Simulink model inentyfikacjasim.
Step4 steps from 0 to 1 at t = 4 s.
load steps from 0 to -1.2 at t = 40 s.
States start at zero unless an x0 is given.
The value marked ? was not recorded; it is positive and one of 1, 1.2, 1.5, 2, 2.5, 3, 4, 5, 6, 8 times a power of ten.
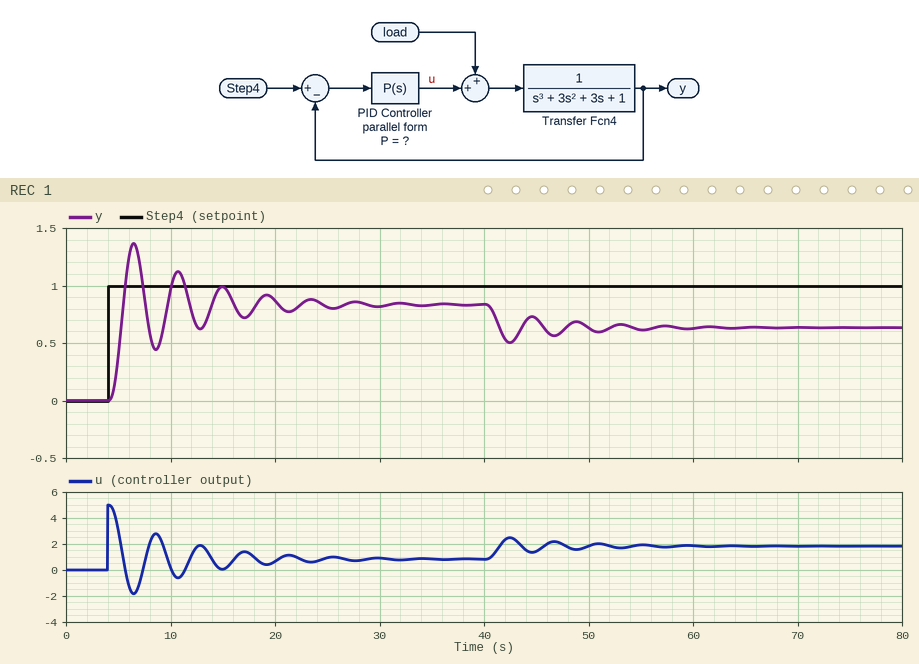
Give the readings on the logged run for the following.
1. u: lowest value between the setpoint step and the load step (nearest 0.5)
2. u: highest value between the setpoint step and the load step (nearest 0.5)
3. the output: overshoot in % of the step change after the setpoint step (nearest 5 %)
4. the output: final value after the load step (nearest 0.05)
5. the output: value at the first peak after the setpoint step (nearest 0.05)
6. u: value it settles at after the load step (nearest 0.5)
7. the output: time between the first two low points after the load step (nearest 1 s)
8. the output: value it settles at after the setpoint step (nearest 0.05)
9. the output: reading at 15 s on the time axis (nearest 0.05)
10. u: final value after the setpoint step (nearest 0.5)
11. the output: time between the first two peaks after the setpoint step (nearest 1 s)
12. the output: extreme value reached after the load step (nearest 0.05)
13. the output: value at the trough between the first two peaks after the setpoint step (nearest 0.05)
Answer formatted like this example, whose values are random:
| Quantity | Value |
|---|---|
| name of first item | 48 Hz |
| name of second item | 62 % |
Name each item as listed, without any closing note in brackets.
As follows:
| Quantity | Value |
|---|---|
| u: lowest value between the setpoint step and the load step | -2.0 |
| u: highest value between the setpoint step and the load step | 5.0 |
| the output: overshoot in % of the step change after the setpoint step | 65 % |
| the output: final value after the load step | 0.65 |
| the output: value at the first peak after the setpoint step | 1.35 |
| u: value it settles at after the load step | 2.0 |
| the output: time between the first two low points after the load step | 4 s |
| the output: value it settles at after the setpoint step | 0.85 |
| the output: reading at 15 s on the time axis | 1.00 |
| u: final value after the setpoint step | 1.0 |
| the output: time between the first two peaks after the setpoint step | 4 s |
| the output: extreme value reached after the load step | 0.50 |
| the output: value at the trough between the first two peaks after the setpoint step | 0.45 |
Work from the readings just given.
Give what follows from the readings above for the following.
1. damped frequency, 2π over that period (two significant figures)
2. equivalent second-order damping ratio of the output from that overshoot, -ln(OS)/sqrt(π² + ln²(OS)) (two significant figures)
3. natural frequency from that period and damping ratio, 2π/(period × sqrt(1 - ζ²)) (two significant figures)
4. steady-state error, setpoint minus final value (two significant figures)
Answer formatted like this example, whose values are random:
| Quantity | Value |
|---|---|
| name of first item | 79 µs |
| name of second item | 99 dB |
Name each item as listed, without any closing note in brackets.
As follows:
| Quantity | Value |
|---|---|
| damped frequency, 2π over that period | 1.6 rad/s |
| equivalent second-order damping ratio of the output from that overshoot, -ln(OS)/sqrt(π² + ln²(OS)) | 0.14 |
| natural frequency from that period and damping ratio, 2π/(period × sqrt(1 - ζ²)) | 1.6 rad/s |
| steady-state error, setpoint minus final value | 0.15 |
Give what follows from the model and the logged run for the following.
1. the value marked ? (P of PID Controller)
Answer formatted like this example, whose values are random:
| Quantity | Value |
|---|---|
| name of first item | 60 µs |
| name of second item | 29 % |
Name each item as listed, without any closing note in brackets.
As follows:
| Quantity | Value |
|---|---|
| the value marked ? | 5 |
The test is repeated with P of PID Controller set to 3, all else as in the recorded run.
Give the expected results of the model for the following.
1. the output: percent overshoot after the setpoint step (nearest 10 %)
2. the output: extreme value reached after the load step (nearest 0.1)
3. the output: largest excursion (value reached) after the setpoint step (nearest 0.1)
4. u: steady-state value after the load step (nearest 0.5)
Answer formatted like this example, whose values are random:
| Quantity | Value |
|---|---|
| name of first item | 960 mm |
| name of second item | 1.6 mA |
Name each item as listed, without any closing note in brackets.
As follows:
| Quantity | Value |
|---|---|
| the output: percent overshoot after the setpoint step | 40 % |
| the output: extreme value reached after the load step | 0.3 |
| the output: largest excursion (value reached) after the setpoint step | 1.1 |
| u: steady-state value after the load step | 1.5 |
